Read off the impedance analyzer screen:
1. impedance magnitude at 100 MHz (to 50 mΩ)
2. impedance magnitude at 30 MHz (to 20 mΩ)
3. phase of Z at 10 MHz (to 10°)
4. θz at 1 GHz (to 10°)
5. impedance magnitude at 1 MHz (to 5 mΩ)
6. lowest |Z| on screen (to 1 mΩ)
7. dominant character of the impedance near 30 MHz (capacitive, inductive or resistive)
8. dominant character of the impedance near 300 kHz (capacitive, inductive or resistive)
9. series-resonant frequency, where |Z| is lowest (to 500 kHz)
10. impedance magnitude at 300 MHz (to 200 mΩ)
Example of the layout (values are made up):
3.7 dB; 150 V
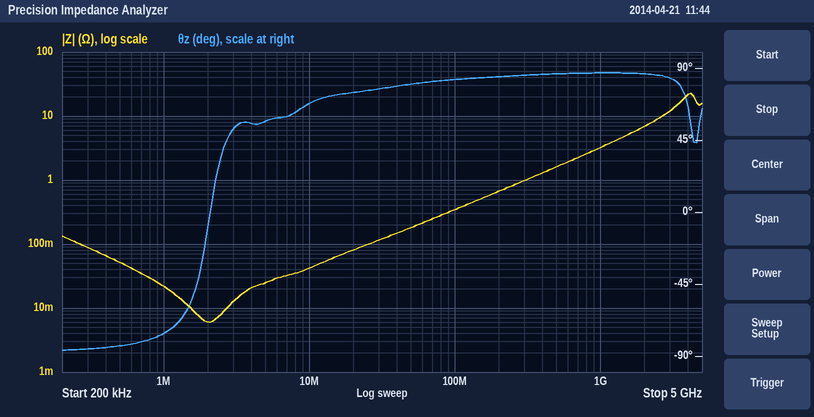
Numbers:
350 mΩ; 120 mΩ; 70°; 90°; 20 mΩ; 6 mΩ; inductive; capacitive; 2.0 MHz; 1.0 Ω
